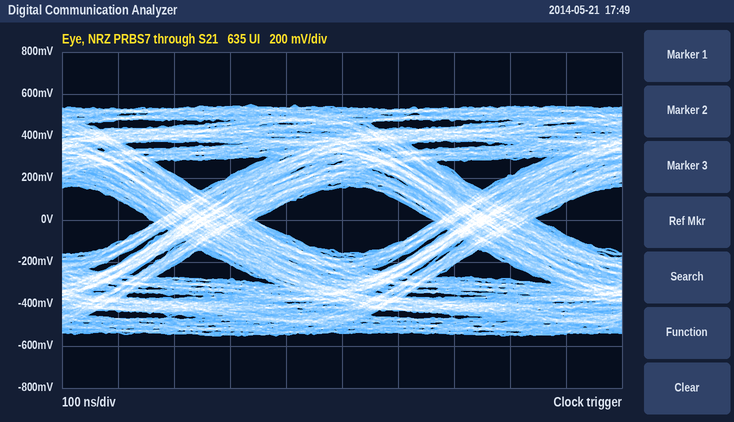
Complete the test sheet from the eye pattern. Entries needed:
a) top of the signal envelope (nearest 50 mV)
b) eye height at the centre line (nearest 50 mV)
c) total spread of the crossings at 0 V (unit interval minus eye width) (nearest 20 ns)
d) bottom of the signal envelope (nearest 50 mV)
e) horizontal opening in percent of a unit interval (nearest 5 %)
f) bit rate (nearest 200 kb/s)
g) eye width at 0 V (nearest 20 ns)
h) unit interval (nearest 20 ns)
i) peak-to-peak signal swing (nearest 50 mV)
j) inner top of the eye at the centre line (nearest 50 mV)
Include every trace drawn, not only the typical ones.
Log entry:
550 mV
300 mV
180 ns
-550 mV
65 %
2.0 Mb/s
320 ns
500 ns
1.10 V
150 mV
